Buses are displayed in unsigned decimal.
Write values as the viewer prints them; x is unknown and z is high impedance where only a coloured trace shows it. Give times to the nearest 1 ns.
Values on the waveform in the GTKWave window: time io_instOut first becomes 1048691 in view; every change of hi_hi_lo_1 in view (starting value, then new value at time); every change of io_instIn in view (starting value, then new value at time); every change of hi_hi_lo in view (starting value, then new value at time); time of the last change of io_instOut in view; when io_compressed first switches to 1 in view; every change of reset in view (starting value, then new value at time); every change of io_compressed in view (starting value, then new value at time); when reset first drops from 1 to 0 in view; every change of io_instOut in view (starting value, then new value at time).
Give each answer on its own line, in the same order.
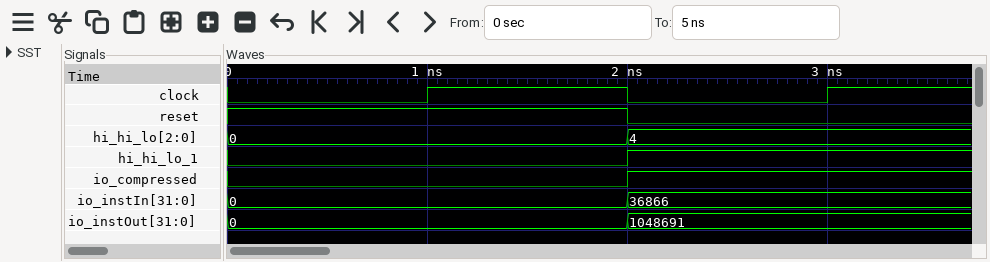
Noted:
2 ns
0, 1 at 2 ns
0, 36866 at 2 ns
0, 4 at 2 ns
2 ns
2 ns
1, 0 at 2 ns
0, 1 at 2 ns
2 ns
0, 1048691 at 2 ns
